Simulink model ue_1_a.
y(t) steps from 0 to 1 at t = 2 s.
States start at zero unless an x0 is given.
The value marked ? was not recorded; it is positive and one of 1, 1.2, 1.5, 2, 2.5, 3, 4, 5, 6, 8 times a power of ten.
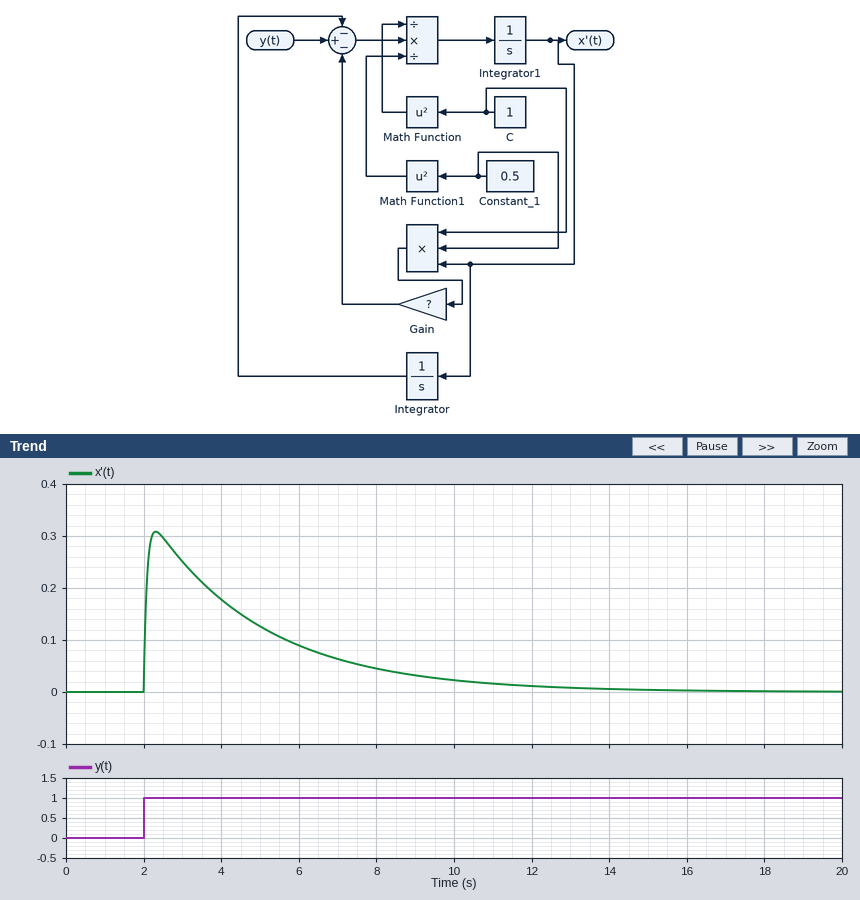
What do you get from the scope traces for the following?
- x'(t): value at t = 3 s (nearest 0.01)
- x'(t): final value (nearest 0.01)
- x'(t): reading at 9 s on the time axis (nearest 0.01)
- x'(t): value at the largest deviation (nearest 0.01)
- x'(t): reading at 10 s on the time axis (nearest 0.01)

0.25
0.00
0.03
0.31
0.02
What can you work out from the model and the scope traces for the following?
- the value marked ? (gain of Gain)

6
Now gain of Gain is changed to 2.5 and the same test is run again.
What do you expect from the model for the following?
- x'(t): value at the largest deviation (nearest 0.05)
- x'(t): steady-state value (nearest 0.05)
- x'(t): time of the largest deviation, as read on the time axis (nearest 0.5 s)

0.65
0.00
2.5 s
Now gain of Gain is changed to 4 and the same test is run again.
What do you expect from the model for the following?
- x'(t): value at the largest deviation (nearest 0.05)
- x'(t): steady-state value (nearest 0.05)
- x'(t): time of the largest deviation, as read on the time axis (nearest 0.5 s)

0.45
0.00
2.5 s
